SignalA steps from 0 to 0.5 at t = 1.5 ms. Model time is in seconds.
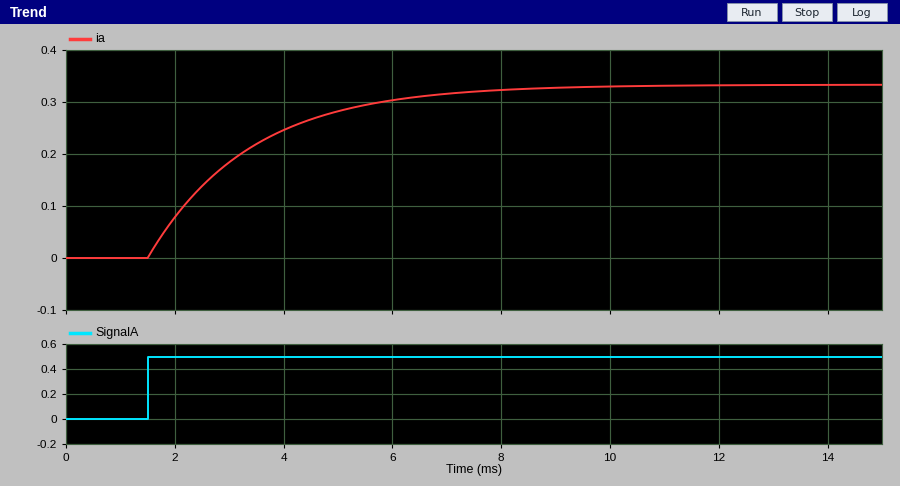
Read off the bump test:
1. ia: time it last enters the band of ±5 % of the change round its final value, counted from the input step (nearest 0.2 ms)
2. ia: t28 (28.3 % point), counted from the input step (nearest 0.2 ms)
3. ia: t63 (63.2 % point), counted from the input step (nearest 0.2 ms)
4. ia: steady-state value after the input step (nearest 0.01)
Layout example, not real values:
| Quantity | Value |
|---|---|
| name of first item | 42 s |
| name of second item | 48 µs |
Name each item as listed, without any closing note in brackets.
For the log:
| Quantity | Value |
|---|---|
| ia: time it last enters the band of ±5 % of the change round its final value, counted from the input step | 5.6 ms |
| ia: t28 (28.3 % point), counted from the input step | 0.6 ms |
| ia: t63 (63.2 % point), counted from the input step | 1.8 ms |
| ia: steady-state value after the input step | 0.33 |
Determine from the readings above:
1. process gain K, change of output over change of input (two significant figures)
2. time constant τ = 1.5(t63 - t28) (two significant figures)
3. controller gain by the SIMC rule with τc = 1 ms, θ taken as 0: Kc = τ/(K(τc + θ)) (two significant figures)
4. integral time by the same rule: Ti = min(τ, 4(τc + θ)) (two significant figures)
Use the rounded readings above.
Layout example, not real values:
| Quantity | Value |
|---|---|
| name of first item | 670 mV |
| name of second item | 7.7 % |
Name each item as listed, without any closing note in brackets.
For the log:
| Quantity | Value |
|---|---|
| process gain K, change of output over change of input | 0.66 |
| time constant τ = 1.5(t63 - t28) | 1.8 ms |
| controller gain by the SIMC rule with τc = 1 ms, θ taken as 0: Kc = τ/(K(τc + θ)) | 2.7 |
| integral time by the same rule: Ti = min(τ, 4(τc + θ)) | 1.8 ms |
